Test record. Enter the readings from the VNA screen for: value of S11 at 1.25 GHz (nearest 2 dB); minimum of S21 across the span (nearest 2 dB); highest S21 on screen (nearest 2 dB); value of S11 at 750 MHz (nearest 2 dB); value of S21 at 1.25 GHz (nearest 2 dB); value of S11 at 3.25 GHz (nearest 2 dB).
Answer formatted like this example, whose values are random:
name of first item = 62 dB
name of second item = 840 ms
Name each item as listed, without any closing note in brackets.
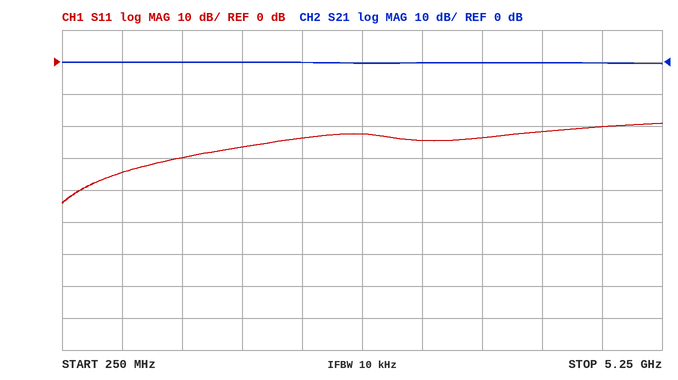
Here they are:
value of S11 at 1.25 GHz = -30 dB
minimum of S21 across the span = 0 dB
highest S21 on screen = 0 dB
value of S11 at 750 MHz = -34 dB
value of S21 at 1.25 GHz = 0 dB
value of S11 at 3.25 GHz = -24 dB
